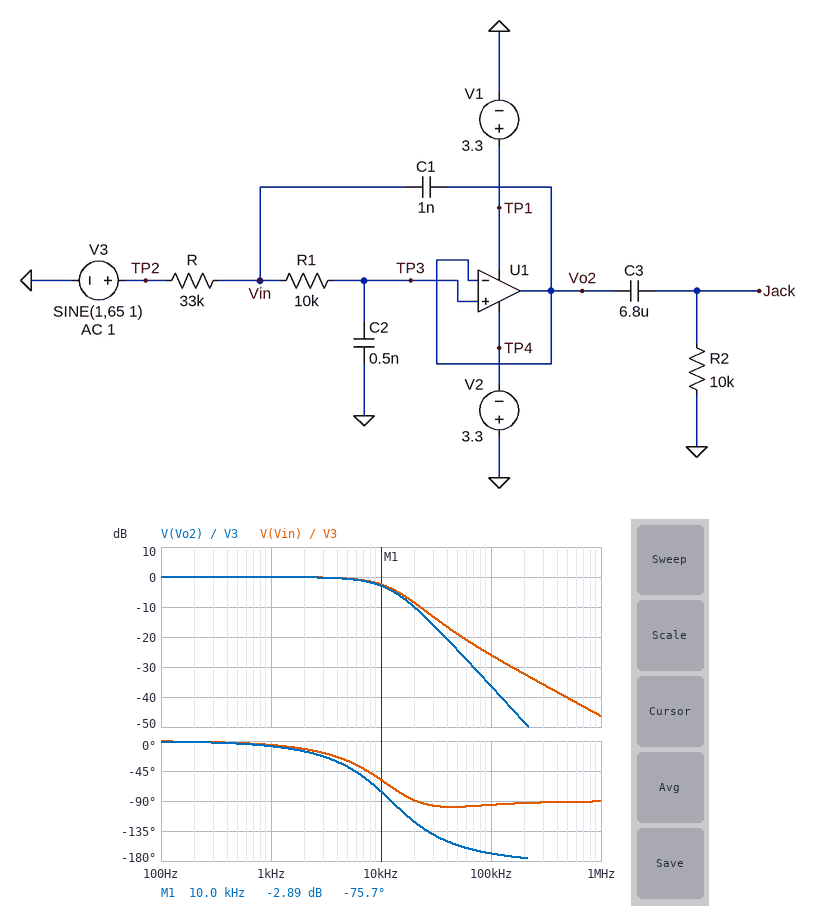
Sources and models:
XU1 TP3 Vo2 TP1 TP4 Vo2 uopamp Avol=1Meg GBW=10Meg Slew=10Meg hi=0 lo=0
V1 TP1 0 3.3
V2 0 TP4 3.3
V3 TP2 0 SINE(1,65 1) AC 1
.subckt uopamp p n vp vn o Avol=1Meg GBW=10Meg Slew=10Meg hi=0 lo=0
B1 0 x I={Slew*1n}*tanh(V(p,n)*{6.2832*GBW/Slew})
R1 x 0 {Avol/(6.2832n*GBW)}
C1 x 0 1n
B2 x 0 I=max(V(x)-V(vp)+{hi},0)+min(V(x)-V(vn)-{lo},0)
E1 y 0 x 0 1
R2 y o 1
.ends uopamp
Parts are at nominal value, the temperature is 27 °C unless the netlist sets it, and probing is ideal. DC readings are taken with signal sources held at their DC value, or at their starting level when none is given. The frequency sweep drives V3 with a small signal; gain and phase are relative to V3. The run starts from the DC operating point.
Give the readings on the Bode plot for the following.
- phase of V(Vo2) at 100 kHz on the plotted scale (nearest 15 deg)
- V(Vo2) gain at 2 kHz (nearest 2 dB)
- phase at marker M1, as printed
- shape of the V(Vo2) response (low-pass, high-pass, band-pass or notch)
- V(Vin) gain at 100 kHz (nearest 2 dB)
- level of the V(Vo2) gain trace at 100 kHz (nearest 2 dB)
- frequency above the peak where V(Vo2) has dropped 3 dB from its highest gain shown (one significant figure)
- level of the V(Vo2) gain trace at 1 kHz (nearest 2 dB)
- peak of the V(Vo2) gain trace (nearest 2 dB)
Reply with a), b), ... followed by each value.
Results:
a) -165 deg
b) 0 dB
c) -75.7 deg
d) low-pass
e) -26 dB
f) -36 dB
g) 10 kHz
h) 0 dB
i) 0 dB
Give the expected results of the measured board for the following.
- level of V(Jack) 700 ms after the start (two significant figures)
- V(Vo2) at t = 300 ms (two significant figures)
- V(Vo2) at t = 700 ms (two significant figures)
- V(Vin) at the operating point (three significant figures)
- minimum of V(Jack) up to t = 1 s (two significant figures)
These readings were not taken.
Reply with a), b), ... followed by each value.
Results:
a) -360 mV
b) 3.3 V
c) -3.3 V
d) 1.00 V
e) -5.9 V
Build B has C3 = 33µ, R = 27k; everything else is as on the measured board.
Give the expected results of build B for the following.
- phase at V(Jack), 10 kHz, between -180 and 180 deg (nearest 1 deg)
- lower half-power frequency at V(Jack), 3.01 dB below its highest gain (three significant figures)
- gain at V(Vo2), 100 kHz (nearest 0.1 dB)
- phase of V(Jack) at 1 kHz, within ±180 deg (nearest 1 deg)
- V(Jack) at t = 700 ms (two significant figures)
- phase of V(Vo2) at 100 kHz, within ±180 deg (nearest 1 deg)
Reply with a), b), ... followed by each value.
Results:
a) -68 deg
b) 482 mHz
c) -34.6 dB
d) -7 deg
e) -3.4 V
f) -168 deg
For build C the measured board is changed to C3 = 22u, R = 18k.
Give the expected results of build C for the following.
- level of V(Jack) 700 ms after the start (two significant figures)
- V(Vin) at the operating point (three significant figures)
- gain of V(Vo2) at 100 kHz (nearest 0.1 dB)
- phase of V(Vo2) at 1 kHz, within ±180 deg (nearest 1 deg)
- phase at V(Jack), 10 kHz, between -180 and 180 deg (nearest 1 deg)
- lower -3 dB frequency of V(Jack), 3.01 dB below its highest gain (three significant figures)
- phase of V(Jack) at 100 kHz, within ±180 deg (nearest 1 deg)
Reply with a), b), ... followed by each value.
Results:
a) -2.6 V
b) 1.00 V
c) -31.1 dB
d) -5 deg
e) -54 deg
f) 723 mHz
g) -166 deg
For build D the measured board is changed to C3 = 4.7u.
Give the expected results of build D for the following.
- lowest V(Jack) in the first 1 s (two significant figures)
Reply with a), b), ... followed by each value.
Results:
a) -5.6 V
